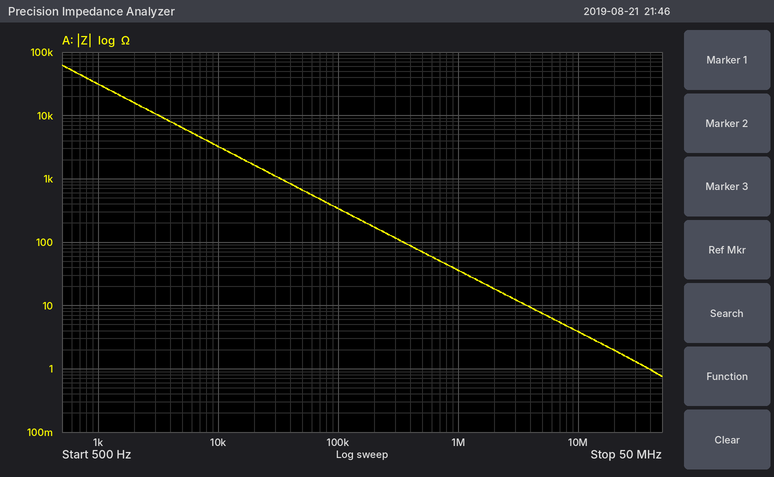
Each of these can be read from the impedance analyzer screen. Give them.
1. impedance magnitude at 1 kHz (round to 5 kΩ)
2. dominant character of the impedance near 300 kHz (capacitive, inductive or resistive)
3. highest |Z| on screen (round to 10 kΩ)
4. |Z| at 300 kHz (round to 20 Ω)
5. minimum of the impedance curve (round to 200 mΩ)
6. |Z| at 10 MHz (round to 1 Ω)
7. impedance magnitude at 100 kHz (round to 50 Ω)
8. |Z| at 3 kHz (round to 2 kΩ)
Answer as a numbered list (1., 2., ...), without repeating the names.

1. 30 kΩ
2. capacitive
3. 60 kΩ
4. 120 Ω
5. 800 mΩ
6. 4 Ω
7. 350 Ω
8. 10 kΩ
